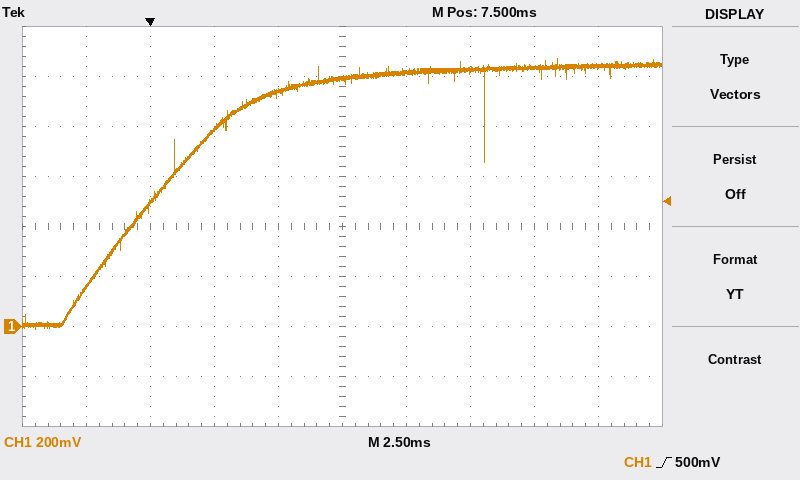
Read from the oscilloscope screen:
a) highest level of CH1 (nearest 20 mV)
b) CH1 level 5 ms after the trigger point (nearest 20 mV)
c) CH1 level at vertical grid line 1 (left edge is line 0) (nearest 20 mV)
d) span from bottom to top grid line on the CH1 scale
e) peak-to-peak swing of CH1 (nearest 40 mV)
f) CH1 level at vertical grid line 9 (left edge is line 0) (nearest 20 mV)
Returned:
1.08 V
940 mV
160 mV
1.6 V
1.08 V
1.04 V
